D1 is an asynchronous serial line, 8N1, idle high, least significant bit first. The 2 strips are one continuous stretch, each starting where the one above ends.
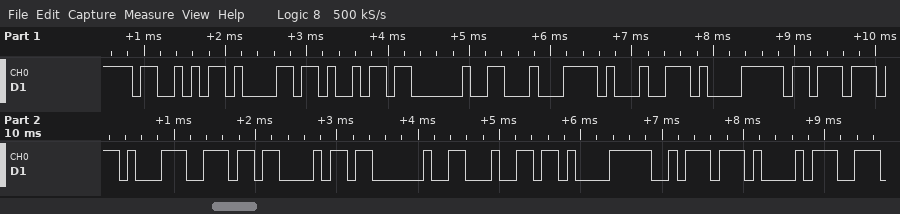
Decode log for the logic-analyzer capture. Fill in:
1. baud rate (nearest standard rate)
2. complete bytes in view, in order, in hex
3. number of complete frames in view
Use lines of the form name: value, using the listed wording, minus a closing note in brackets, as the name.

baud rate: 9600 baud
complete bytes in view, in order, in hex: 53 61 69 20 C4 91 E1 BB 8B 6E 68 20 64 E1 BA A1
number of complete frames in view: 16
